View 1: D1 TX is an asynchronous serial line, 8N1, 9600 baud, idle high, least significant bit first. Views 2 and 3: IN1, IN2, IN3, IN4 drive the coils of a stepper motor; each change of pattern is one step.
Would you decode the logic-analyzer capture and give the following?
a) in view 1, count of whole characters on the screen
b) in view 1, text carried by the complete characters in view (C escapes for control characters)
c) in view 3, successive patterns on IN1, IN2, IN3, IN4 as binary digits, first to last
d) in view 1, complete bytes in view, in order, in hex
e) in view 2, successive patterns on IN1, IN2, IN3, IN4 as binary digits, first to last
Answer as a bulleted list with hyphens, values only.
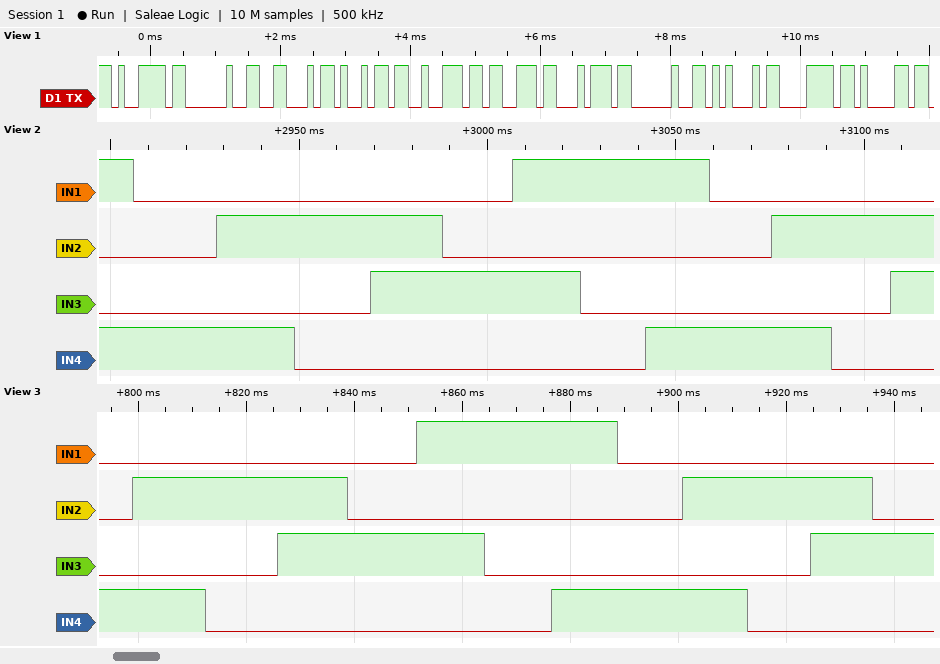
- 11
- "y First Exa"
- 0001 0101 0100 0110 0010 1010 1000 1001 0001 0101 0100 0110 0010
- 0x79 0x20 0x46 0x69 0x72 0x73 0x74 0x20 0x45 0x78 0x61
- 1001 0001 0101 0100 0110 0010 1010 1000 1001 0001 0101 0100 0110
